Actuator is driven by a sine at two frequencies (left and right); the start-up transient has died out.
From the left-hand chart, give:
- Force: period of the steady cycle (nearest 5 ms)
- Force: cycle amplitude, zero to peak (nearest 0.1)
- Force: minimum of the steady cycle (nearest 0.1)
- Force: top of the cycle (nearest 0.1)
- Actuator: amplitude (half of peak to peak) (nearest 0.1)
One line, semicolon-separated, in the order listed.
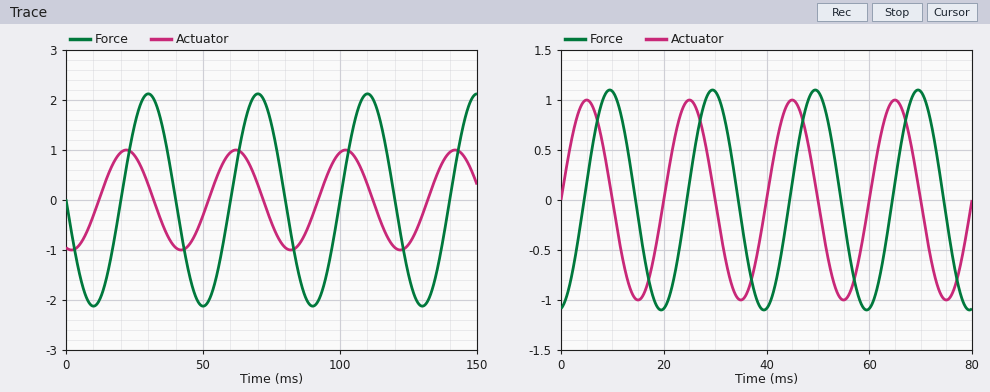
40 ms; 2.1; -2.1; 2.1; 1.0
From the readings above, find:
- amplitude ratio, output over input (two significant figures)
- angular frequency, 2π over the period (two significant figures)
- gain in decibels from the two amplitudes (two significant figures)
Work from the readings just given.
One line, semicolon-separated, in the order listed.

2.1; 0.16 rad/ms; 6.4 dB
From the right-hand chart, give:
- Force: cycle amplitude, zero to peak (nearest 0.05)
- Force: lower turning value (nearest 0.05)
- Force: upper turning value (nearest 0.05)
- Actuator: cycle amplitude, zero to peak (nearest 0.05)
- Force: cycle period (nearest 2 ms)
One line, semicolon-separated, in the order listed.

1.10; -1.10; 1.10; 1.00; 20 ms
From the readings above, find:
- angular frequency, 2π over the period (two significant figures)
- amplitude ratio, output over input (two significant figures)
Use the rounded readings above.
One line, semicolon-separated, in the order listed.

0.31 rad/ms; 1.1
